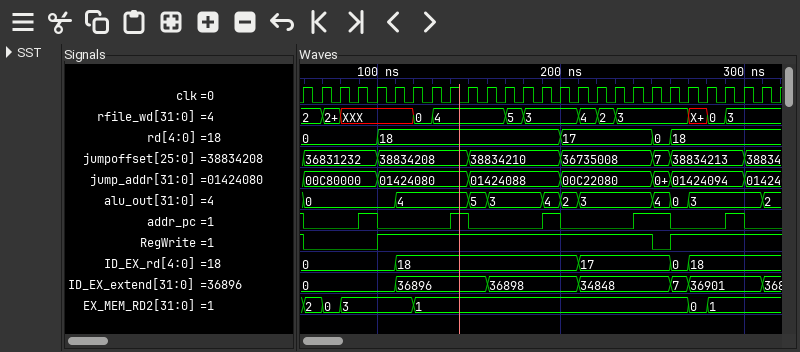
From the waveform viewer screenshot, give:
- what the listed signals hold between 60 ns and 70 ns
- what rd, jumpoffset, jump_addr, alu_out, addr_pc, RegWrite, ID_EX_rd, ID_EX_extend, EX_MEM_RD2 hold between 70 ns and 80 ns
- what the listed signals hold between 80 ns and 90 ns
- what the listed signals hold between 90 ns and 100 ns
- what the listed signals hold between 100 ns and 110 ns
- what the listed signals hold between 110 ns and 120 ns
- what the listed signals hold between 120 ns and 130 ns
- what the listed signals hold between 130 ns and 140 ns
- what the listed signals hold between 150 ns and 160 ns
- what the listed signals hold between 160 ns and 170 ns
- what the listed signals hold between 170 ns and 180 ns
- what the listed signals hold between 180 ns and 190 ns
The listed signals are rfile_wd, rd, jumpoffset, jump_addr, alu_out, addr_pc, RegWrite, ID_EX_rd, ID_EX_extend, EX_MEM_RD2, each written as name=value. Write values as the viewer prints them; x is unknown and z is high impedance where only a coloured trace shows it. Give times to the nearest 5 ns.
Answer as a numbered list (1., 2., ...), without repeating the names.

1. rfile_wd=2, rd=0, jumpoffset=36831232, jump_addr=00C80000, alu_out=0, addr_pc=0, RegWrite=0, ID_EX_rd=0, ID_EX_extend=0, EX_MEM_RD2=2
2. rd=0, jumpoffset=36831232, jump_addr=00C80000, alu_out=0, addr_pc=0, RegWrite=0, ID_EX_rd=0, ID_EX_extend=0, EX_MEM_RD2=0
3. rfile_wd=XXX, rd=0, jumpoffset=36831232, jump_addr=00C80000, alu_out=0, addr_pc=0, RegWrite=0, ID_EX_rd=0, ID_EX_extend=0, EX_MEM_RD2=3
4. rfile_wd=XXX, rd=0, jumpoffset=36831232, jump_addr=00C80000, alu_out=0, addr_pc=1, RegWrite=0, ID_EX_rd=0, ID_EX_extend=0, EX_MEM_RD2=3
5. rfile_wd=XXX, rd=18, jumpoffset=38834208, jump_addr=01424080, alu_out=0, addr_pc=0, RegWrite=1, ID_EX_rd=0, ID_EX_extend=0, EX_MEM_RD2=3
6. rfile_wd=XXX, rd=18, jumpoffset=38834208, jump_addr=01424080, alu_out=4, addr_pc=0, RegWrite=1, ID_EX_rd=18, ID_EX_extend=36896, EX_MEM_RD2=3
7. rfile_wd=0, rd=18, jumpoffset=38834208, jump_addr=01424080, alu_out=4, addr_pc=0, RegWrite=1, ID_EX_rd=18, ID_EX_extend=36896, EX_MEM_RD2=1
8. rfile_wd=4, rd=18, jumpoffset=38834208, jump_addr=01424080, alu_out=4, addr_pc=0, RegWrite=1, ID_EX_rd=18, ID_EX_extend=36896, EX_MEM_RD2=1
9. rfile_wd=4, rd=18, jumpoffset=38834210, jump_addr=01424088, alu_out=5, addr_pc=0, RegWrite=1, ID_EX_rd=18, ID_EX_extend=36896, EX_MEM_RD2=1
10. rfile_wd=4, rd=18, jumpoffset=38834210, jump_addr=01424088, alu_out=3, addr_pc=0, RegWrite=1, ID_EX_rd=18, ID_EX_extend=36898, EX_MEM_RD2=1
11. rfile_wd=5, rd=18, jumpoffset=38834210, jump_addr=01424088, alu_out=3, addr_pc=0, RegWrite=1, ID_EX_rd=18, ID_EX_extend=36898, EX_MEM_RD2=1
12. rfile_wd=3, rd=18, jumpoffset=38834210, jump_addr=01424088, alu_out=3, addr_pc=0, RegWrite=1, ID_EX_rd=18, ID_EX_extend=36898, EX_MEM_RD2=1
